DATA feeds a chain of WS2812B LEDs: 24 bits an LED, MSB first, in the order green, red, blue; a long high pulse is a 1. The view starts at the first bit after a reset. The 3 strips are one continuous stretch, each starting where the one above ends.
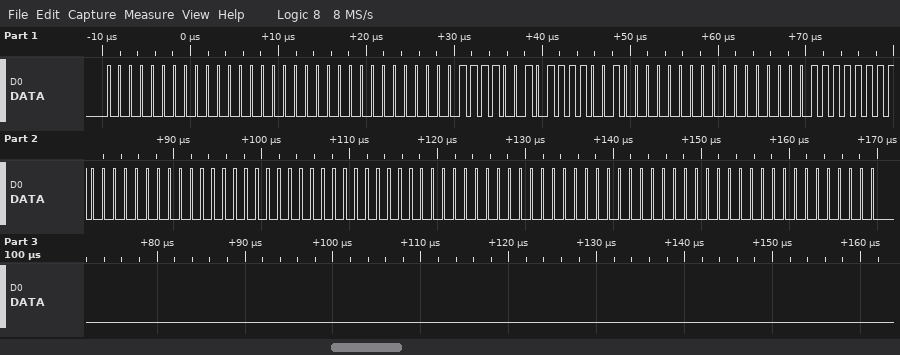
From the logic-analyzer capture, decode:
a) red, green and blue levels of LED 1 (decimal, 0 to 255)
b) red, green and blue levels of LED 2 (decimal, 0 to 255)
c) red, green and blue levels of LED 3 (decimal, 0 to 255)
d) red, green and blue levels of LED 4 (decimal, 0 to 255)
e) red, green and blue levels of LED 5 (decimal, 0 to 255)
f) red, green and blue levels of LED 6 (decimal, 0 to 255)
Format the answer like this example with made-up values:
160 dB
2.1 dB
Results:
0, 0, 0
242, 0, 242
0, 0, 255
0, 0, 0
0, 0, 0
0, 0, 0
